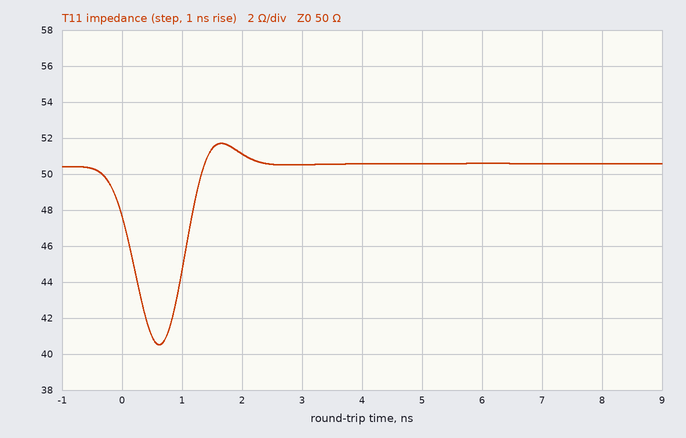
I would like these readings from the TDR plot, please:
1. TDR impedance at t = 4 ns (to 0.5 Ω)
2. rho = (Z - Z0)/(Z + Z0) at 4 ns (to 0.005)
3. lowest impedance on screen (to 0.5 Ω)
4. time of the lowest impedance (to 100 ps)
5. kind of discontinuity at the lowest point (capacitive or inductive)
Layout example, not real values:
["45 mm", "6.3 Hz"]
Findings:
["50.5 Ω", "+0.005", "40.5 Ω", "600 ps", "capacitive"]
